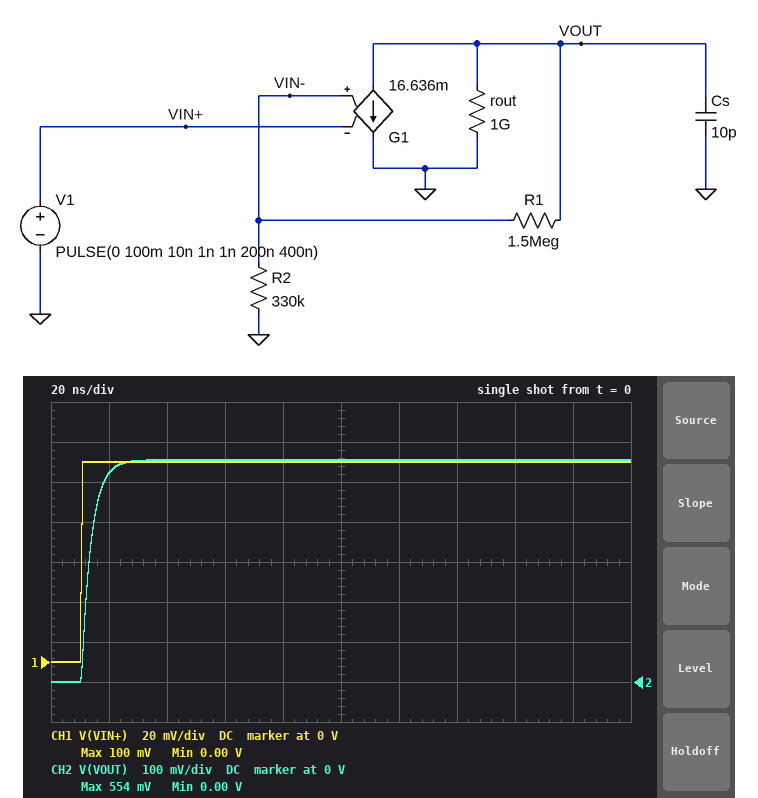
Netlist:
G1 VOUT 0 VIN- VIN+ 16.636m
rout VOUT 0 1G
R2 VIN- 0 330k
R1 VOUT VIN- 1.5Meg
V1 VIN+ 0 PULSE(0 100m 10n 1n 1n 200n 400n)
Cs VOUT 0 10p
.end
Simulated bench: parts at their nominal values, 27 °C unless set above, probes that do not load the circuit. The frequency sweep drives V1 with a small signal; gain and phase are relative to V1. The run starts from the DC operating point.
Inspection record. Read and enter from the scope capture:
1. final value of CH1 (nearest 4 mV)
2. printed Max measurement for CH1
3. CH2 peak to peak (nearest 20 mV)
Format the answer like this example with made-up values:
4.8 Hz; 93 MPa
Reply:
100 mV; 100 mV; 560 mV
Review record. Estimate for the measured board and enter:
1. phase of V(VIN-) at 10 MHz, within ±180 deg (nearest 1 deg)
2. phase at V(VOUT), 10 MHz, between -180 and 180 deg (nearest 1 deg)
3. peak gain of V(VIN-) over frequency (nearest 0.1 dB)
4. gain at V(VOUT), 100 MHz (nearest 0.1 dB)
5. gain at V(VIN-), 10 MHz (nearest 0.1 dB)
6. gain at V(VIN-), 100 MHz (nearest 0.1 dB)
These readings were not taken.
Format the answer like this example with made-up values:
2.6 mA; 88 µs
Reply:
-12 deg; -12 deg; 0 dB; 7.6 dB; -0.2 dB; -7.3 dB
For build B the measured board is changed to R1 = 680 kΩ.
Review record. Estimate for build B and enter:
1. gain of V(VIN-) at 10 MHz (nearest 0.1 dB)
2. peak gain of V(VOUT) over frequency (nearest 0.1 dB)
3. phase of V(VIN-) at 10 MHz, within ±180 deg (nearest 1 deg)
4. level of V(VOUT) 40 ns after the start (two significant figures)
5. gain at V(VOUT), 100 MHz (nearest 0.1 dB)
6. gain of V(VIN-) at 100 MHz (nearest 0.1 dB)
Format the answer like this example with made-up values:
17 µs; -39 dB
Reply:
-0.1 dB; 9.7 dB; -7 deg; 310 mV; 6.0 dB; -3.7 dB
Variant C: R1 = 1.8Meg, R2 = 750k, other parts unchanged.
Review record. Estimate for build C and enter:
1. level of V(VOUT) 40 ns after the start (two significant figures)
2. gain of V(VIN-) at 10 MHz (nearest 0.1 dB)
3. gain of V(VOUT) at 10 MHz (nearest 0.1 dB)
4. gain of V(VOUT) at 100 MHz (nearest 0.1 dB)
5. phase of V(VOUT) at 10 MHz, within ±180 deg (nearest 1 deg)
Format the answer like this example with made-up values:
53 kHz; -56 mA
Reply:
340 mV; -0.1 dB; 10.6 dB; 6.4 dB; -7 deg
